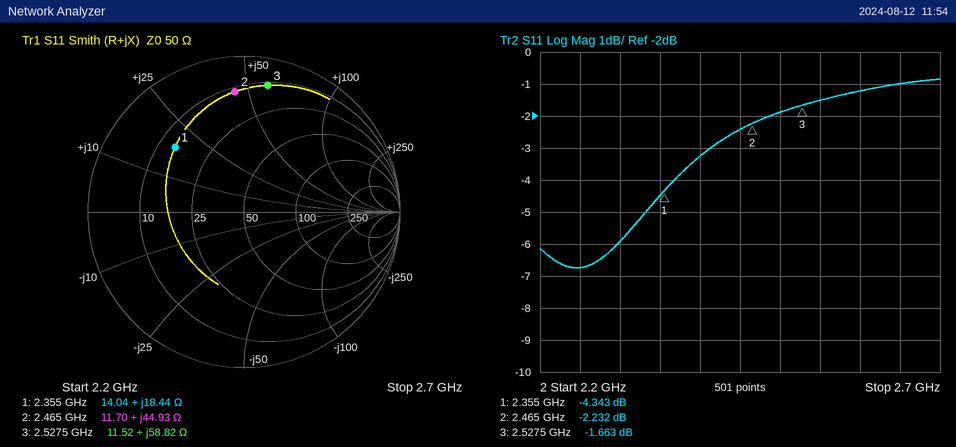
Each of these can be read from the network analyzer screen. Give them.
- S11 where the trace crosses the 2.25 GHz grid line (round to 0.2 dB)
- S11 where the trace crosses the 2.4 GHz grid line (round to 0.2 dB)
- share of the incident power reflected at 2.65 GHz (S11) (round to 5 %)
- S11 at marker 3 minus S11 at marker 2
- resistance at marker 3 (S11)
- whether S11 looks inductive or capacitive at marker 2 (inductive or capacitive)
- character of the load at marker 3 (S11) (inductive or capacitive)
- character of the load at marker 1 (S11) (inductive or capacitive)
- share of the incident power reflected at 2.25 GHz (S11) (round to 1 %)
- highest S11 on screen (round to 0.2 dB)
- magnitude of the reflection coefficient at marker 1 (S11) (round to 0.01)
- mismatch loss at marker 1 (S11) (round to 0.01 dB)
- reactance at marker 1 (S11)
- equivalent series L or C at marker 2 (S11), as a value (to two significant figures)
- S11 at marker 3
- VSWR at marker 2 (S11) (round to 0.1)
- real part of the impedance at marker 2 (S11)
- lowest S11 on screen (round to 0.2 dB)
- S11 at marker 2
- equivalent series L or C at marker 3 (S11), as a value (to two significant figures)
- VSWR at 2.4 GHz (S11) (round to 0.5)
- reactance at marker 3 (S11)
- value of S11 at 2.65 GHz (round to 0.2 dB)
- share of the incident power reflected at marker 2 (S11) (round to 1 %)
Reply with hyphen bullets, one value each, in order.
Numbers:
- -6.8 dB
- -3.2 dB
- 80 %
- 0.569 dB
- 11.52 Ω
- inductive
- inductive
- inductive
- 21 %
- -0.8 dB
- 0.61
- 1.99 dB
- +18.44 Ω
- 2.9 nH
- -1.663 dB
- 7.8
- 11.70 Ω
- -6.8 dB
- -2.232 dB
- 3.7 nH
- 5.5
- +58.82 Ω
- -1.0 dB
- 60 %
